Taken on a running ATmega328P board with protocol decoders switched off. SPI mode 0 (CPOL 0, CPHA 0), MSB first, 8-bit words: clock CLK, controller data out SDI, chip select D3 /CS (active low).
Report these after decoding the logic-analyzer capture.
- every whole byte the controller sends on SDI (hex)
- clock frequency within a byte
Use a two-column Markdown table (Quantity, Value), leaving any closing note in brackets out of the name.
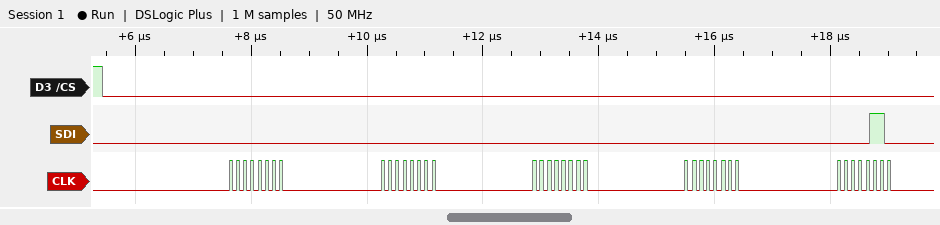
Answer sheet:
| Quantity | Value |
|---|---|
| every whole byte the controller sends on SDI | 0x00 0x00 0x00 0x00 0x06 |
| clock frequency within a byte | 8 MHz |
